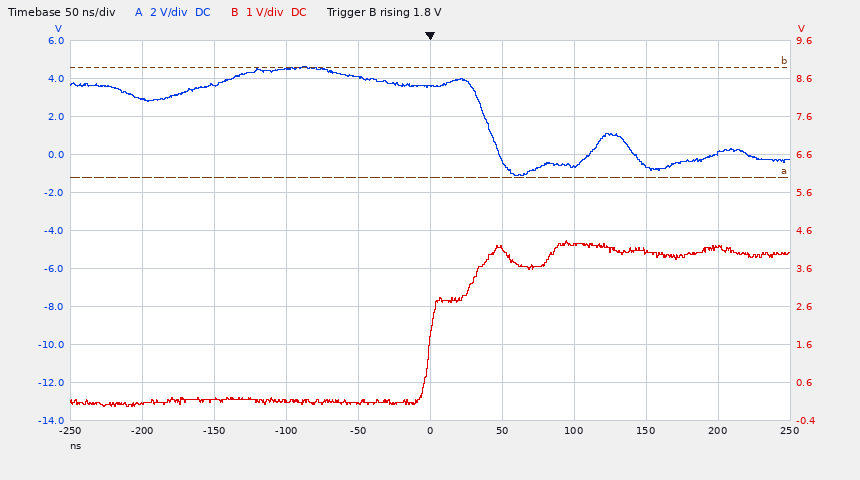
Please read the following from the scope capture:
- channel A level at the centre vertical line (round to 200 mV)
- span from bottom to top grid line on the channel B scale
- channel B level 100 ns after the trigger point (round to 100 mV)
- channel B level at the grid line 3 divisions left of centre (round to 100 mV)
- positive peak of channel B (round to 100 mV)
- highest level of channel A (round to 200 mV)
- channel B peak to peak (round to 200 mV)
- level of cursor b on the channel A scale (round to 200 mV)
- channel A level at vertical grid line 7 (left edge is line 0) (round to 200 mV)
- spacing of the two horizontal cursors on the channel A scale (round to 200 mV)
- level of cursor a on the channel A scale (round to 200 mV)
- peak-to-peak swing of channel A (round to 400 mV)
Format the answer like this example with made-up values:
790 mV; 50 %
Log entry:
3.6 V; 10 V; 4.2 V; 200 mV; 4.3 V; 4.6 V; 4.4 V; 4.6 V; -600 mV; 5.8 V; -1.2 V; 5.6 V
